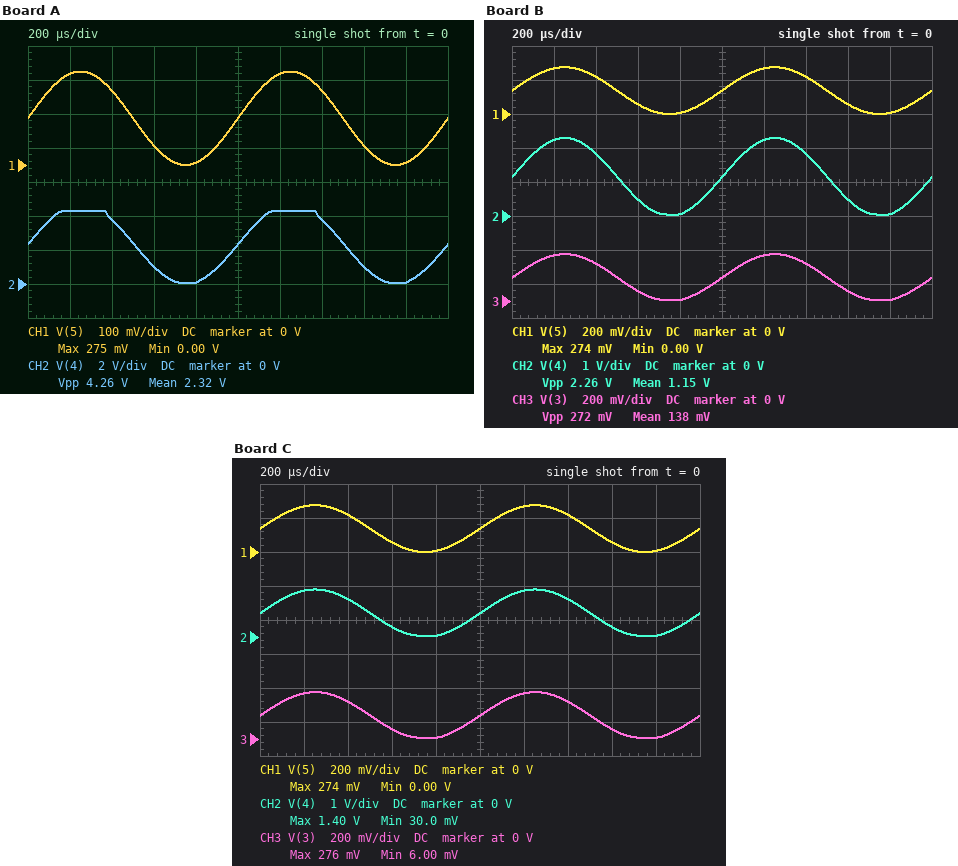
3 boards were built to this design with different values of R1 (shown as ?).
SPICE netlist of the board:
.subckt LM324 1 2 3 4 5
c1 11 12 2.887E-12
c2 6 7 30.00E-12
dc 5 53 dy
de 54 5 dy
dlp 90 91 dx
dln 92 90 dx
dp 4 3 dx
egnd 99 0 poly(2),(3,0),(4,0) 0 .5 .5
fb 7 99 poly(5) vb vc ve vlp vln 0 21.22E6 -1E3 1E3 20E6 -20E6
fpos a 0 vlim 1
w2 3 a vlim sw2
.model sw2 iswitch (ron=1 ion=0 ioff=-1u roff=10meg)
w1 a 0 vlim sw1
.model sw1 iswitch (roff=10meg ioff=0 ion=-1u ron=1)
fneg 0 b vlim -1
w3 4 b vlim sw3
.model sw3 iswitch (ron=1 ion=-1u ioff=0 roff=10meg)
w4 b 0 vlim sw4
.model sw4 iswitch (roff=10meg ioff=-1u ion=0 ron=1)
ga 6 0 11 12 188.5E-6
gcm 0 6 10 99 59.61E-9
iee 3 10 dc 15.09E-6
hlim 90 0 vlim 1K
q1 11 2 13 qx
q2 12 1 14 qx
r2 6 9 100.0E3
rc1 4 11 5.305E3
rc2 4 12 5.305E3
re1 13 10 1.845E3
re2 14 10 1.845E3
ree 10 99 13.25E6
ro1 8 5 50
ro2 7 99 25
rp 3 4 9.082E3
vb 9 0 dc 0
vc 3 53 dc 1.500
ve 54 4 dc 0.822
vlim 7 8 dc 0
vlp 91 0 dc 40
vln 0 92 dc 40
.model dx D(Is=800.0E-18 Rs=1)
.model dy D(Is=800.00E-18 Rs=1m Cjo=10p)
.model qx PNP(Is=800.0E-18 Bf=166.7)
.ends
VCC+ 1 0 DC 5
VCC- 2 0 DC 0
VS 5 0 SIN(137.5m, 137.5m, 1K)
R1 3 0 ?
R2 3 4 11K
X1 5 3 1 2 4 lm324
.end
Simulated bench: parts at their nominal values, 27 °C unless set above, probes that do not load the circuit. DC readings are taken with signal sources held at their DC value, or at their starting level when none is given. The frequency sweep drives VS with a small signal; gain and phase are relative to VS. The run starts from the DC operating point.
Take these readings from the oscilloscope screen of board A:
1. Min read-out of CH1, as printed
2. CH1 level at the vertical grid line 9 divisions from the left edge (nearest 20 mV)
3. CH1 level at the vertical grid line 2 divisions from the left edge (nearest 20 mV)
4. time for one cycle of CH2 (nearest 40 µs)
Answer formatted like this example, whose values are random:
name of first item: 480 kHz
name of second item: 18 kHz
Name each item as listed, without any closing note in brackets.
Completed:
Min read-out of CH1, as printed: 0.00 V
CH1 level at the vertical grid line 9 divisions from the left edge: 0 V
CH1 level at the vertical grid line 2 divisions from the left edge: 220 mV
time for one cycle of CH2: 1.00 ms
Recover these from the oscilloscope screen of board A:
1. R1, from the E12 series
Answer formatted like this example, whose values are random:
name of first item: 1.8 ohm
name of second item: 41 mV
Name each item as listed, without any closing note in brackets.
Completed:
R1, from the E12 series: 680 Ω
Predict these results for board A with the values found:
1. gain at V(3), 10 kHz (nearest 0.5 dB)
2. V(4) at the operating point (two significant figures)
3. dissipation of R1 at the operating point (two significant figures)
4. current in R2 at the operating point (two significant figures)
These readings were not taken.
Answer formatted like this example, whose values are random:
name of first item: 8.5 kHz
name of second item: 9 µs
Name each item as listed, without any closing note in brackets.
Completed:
gain at V(3), 10 kHz: 0 dB
V(4) at the operating point: 2.4 V
dissipation of R1 at the operating point: 28 µW
current in R2 at the operating point: 200 µA
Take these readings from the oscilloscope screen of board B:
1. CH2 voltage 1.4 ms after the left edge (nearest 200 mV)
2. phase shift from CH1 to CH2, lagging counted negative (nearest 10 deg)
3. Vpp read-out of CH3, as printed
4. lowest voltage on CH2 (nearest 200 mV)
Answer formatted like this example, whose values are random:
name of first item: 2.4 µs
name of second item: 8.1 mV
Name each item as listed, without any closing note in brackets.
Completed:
CH2 voltage 1.4 ms after the left edge: 1.8 V
phase shift from CH1 to CH2, lagging counted negative: 0 deg
Vpp read-out of CH3, as printed: 272 mV
lowest voltage on CH2: 0 V
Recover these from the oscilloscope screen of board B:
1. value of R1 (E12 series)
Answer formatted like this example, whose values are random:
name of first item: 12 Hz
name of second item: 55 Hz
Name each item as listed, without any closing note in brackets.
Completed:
value of R1: 1.5 kΩ
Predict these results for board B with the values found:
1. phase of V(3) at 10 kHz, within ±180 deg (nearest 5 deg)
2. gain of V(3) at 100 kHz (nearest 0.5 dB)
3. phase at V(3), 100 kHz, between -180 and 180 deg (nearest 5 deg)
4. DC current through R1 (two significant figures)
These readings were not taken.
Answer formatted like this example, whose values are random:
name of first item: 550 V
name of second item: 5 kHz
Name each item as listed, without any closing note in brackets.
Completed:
phase of V(3) at 10 kHz, within ±180 deg: -5 deg
gain of V(3) at 100 kHz: -2.0 dB
phase at V(3), 100 kHz, between -180 and 180 deg: -40 deg
DC current through R1: 92 µA
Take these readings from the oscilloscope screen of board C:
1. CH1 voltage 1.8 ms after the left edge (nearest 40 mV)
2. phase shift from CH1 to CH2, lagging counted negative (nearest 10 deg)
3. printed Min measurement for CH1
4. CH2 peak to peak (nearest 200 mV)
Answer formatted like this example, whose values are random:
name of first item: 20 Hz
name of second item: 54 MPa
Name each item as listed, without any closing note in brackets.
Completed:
CH1 voltage 1.8 ms after the left edge: 0 V
phase shift from CH1 to CH2, lagging counted negative: 0 deg
printed Min measurement for CH1: 0.00 V
CH2 peak to peak: 1.4 V
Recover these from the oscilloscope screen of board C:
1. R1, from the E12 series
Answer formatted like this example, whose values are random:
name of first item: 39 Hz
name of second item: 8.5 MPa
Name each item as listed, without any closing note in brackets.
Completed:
R1, from the E12 series: 2.7 kΩ
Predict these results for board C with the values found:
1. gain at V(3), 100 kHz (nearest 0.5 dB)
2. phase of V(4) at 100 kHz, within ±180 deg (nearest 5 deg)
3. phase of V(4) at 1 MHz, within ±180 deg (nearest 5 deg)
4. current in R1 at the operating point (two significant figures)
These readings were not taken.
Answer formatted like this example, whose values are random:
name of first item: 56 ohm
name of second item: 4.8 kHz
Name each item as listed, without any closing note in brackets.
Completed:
gain at V(3), 100 kHz: -1.0 dB
phase of V(4) at 100 kHz, within ±180 deg: -25 deg
phase of V(4) at 1 MHz, within ±180 deg: -90 deg
current in R1 at the operating point: 51 µA
